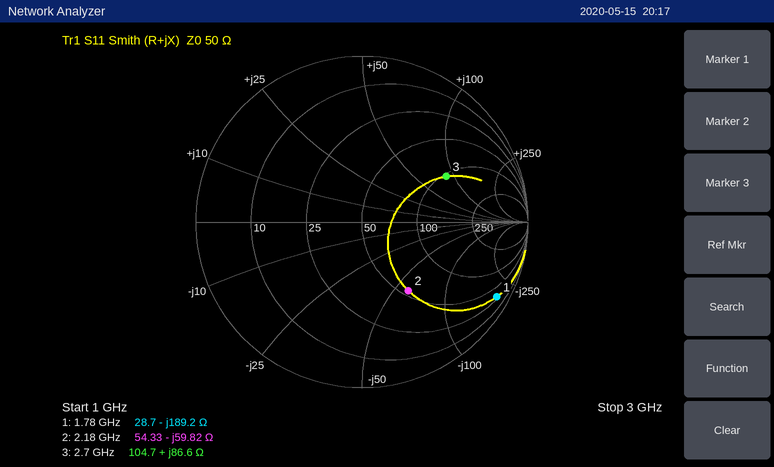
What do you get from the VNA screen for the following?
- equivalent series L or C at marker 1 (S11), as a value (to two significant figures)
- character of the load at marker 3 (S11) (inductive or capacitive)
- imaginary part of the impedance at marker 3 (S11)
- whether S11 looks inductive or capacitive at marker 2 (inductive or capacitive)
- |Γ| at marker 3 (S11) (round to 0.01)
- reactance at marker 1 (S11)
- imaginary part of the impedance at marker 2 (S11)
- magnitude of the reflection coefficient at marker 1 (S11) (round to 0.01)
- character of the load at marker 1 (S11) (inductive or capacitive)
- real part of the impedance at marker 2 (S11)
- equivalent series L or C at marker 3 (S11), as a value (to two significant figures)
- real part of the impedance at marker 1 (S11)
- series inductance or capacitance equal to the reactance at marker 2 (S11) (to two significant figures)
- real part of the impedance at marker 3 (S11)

470 fF
inductive
+86.6 Ω
capacitive
0.58
-189.2 Ω
-59.82 Ω
0.93
capacitive
54.33 Ω
5.1 nH
28.7 Ω
1.2 pF
104.7 Ω
